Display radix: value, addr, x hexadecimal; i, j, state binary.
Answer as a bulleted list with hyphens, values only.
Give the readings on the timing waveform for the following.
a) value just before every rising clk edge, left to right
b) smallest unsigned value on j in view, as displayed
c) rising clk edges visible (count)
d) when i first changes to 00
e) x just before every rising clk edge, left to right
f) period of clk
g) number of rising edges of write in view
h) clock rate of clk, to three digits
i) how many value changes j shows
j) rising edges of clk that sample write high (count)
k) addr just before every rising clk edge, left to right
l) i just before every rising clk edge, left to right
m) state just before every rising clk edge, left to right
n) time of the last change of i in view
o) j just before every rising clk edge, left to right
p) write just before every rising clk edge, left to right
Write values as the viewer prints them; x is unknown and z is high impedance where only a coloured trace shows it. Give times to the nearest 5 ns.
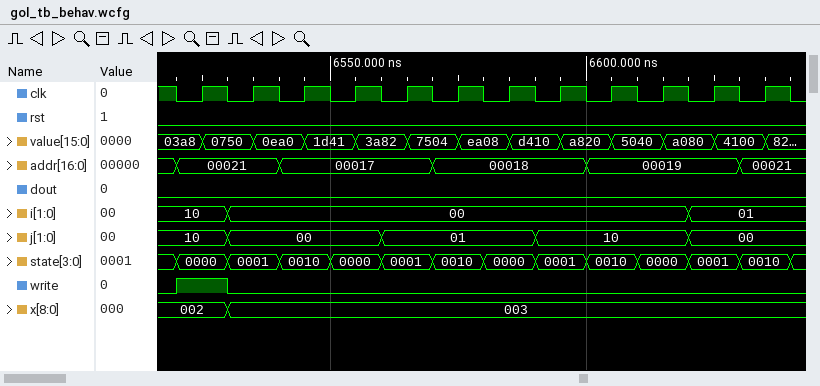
- 03a8, 0750, 0ea0, 1d41, 3a82, 7504, ea08, d410, a820, 5040, a080, 4100
- 00
- 12
- 6530 ns
- 002, 003, 003, 003, 003, 003, 003, 003, 003, 003, 003, 003
- 10 ns
- 1
- 100 MHz
- 4
- 1
- 00021, 00021, 00017, 00017, 00017, 00018, 00018, 00018, 00019, 00019, 00019, 00021
- 10, 00, 00, 00, 00, 00, 00, 00, 00, 00, 01, 01
- 0000, 0001, 0010, 0000, 0001, 0010, 0000, 0001, 0010, 0000, 0001, 0010
- 6620 ns
- 10, 00, 00, 00, 01, 01, 01, 10, 10, 10, 00, 00
- 1 0 0 0 0 0 0 0 0 0 0 0
